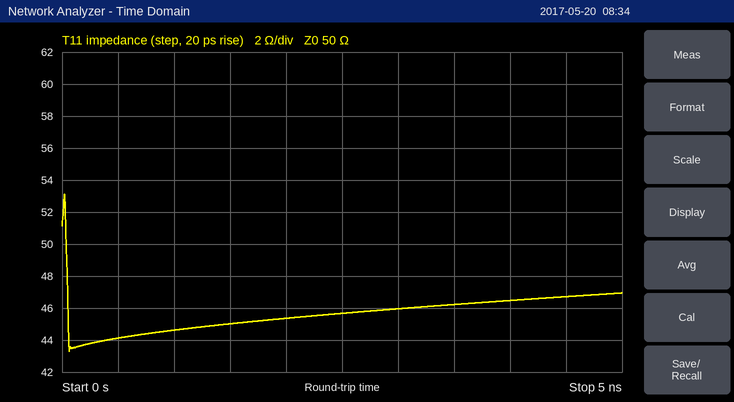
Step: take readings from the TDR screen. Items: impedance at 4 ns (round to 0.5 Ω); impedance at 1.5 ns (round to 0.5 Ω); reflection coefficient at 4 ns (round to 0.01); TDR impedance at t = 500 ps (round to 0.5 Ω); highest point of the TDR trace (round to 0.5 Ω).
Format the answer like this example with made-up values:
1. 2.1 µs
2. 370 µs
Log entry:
1. 46.5 Ω
2. 45.0 Ω
3. -0.04
4. 44.0 Ω
5. 53.0 Ω
